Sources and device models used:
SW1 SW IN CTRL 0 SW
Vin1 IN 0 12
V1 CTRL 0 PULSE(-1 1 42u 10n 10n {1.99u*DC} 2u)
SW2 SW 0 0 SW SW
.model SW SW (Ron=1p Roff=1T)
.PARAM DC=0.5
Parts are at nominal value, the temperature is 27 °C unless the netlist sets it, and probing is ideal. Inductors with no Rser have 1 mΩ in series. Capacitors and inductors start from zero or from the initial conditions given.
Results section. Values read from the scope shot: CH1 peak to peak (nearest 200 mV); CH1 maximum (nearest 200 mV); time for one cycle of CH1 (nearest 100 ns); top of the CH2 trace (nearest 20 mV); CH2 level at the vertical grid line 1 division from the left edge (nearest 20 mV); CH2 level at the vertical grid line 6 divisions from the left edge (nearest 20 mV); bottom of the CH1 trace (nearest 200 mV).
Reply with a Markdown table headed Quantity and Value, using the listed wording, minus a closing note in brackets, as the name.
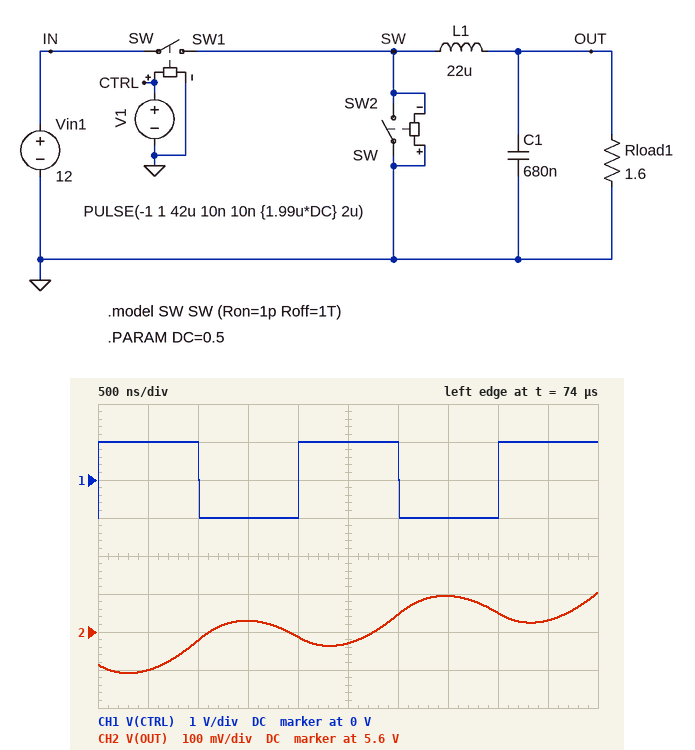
| Quantity | Value |
|---|---|
| CH1 peak to peak | 2.0 V |
| CH1 maximum | 1.0 V |
| time for one cycle of CH1 | 2.0 µs |
| top of the CH2 trace | 5.70 V |
| CH2 level at the vertical grid line 1 division from the left edge | 5.50 V |
| CH2 level at the vertical grid line 6 divisions from the left edge | 5.64 V |
| bottom of the CH1 trace | -1.0 V |
